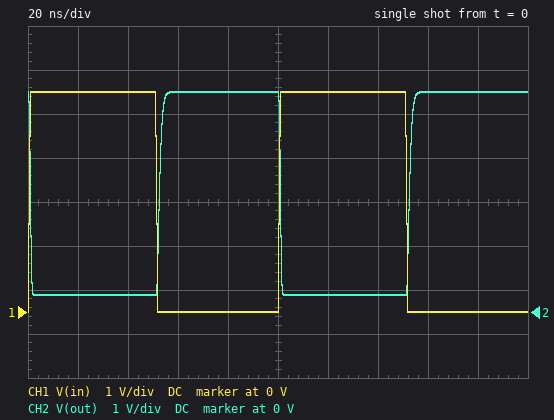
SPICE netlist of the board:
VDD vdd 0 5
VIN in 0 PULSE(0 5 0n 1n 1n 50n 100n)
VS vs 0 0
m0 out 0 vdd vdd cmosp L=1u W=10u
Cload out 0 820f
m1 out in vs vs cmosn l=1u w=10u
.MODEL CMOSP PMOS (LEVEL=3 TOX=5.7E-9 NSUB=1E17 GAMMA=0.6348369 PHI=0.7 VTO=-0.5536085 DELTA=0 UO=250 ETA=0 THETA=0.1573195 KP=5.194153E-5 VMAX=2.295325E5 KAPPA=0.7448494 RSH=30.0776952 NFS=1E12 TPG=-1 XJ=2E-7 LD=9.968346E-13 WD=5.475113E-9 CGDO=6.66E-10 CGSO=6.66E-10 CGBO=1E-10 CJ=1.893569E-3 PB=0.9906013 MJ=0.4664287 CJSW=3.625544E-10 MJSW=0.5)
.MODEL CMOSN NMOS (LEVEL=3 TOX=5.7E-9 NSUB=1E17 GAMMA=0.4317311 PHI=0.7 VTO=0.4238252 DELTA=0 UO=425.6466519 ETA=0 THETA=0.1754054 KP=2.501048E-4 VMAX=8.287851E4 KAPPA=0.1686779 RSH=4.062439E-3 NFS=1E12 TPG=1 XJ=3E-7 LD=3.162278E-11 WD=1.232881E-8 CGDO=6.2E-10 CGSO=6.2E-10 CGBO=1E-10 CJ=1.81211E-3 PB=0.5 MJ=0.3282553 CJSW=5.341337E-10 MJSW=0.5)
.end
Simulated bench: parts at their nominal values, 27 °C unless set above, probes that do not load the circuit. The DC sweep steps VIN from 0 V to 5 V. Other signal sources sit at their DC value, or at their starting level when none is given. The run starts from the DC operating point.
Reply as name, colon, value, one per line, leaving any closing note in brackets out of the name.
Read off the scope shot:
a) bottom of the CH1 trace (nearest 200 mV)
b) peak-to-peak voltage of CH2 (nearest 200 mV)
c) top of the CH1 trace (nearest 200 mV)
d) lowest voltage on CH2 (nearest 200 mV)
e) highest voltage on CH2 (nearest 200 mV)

bottom of the CH1 trace: 0 V
peak-to-peak voltage of CH2: 4.6 V
top of the CH1 trace: 5.0 V
lowest voltage on CH2: 400 mV
highest voltage on CH2: 5.0 V
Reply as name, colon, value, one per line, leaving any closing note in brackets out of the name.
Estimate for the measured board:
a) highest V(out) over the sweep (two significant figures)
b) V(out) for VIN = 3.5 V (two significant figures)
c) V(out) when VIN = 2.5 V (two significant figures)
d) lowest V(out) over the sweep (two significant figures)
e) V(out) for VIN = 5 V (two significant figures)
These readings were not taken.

highest V(out) over the sweep: 5.0 V
V(out) for VIN = 3.5 V: 550 mV
V(out) when VIN = 2.5 V: 1.0 V
lowest V(out) over the sweep: 380 mV
V(out) for VIN = 5 V: 380 mV
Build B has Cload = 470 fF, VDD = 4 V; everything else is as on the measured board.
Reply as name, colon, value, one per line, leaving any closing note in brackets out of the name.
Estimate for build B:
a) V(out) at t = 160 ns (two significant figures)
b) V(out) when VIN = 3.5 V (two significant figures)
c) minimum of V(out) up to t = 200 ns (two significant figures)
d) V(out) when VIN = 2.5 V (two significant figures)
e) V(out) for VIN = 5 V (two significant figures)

V(out) at t = 160 ns: 4.0 V
V(out) when VIN = 3.5 V: 340 mV
minimum of V(out) up to t = 200 ns: 230 mV
V(out) when VIN = 2.5 V: 510 mV
V(out) for VIN = 5 V: 250 mV
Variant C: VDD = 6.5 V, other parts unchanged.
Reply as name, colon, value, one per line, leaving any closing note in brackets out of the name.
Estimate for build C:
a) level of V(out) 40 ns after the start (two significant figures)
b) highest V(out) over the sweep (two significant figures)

level of V(out) 40 ns after the start: 640 mV
highest V(out) over the sweep: 6.5 V
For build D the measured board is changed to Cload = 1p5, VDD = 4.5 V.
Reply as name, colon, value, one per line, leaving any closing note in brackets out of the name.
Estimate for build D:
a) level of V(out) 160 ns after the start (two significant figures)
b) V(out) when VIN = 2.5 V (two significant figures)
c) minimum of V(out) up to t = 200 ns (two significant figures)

level of V(out) 160 ns after the start: 4.5 V
V(out) when VIN = 2.5 V: 710 mV
minimum of V(out) up to t = 200 ns: 310 mV
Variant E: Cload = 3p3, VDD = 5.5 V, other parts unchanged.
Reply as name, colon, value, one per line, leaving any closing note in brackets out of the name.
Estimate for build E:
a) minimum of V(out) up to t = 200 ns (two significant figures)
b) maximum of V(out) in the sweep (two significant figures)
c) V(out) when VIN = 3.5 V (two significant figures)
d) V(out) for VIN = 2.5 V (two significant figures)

minimum of V(out) up to t = 200 ns: 460 mV
maximum of V(out) in the sweep: 5.5 V
V(out) when VIN = 3.5 V: 680 mV
V(out) for VIN = 2.5 V: 2.5 V
